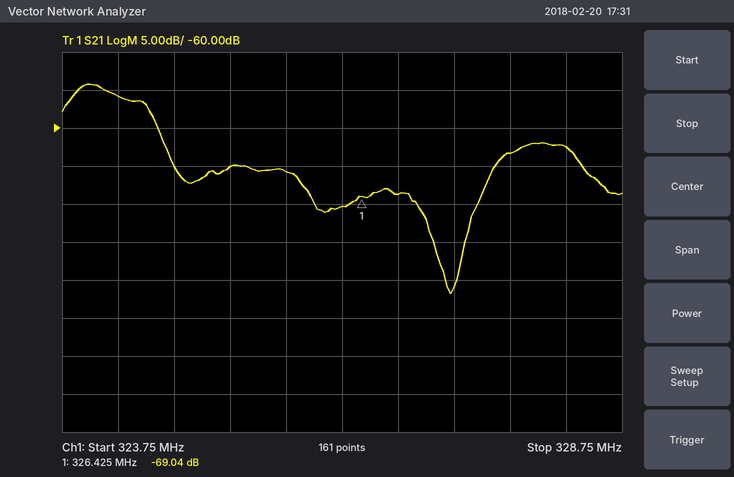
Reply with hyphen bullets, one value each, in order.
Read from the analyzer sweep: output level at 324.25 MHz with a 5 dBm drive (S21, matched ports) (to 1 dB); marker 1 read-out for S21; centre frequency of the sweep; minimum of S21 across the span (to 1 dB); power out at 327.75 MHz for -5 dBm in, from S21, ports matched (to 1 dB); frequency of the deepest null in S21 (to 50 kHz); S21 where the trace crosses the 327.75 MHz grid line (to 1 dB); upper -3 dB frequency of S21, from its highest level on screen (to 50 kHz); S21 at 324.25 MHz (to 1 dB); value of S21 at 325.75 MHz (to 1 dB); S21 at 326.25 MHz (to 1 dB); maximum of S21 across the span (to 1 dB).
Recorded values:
- -51 dBm
- -69.04 dB
- 326.25 MHz
- -82 dB
- -68 dBm
- 327.20 MHz
- -63 dB
- 324.50 MHz
- -56 dB
- -66 dB
- -70 dB
- -54 dB
